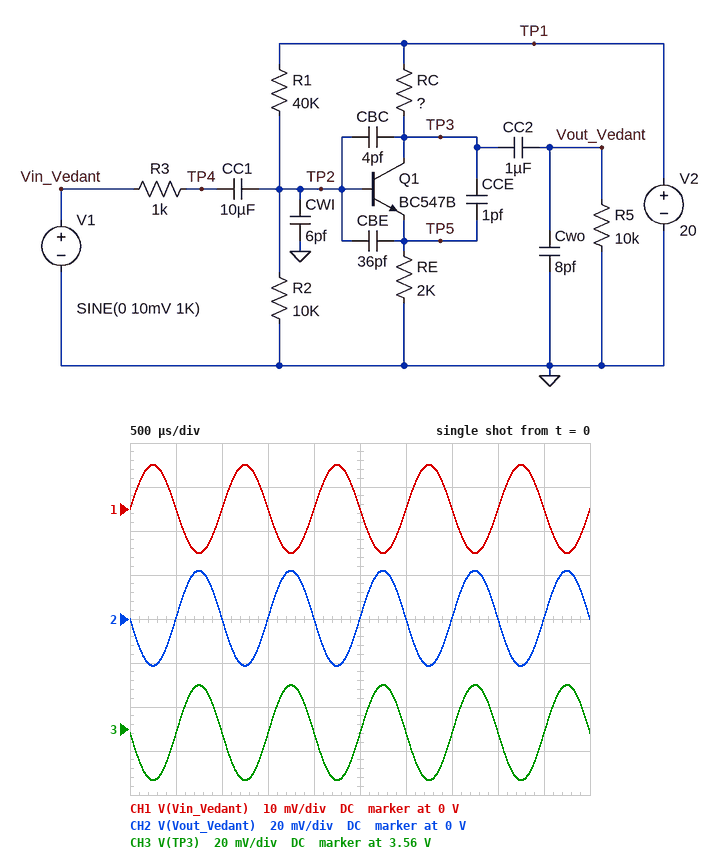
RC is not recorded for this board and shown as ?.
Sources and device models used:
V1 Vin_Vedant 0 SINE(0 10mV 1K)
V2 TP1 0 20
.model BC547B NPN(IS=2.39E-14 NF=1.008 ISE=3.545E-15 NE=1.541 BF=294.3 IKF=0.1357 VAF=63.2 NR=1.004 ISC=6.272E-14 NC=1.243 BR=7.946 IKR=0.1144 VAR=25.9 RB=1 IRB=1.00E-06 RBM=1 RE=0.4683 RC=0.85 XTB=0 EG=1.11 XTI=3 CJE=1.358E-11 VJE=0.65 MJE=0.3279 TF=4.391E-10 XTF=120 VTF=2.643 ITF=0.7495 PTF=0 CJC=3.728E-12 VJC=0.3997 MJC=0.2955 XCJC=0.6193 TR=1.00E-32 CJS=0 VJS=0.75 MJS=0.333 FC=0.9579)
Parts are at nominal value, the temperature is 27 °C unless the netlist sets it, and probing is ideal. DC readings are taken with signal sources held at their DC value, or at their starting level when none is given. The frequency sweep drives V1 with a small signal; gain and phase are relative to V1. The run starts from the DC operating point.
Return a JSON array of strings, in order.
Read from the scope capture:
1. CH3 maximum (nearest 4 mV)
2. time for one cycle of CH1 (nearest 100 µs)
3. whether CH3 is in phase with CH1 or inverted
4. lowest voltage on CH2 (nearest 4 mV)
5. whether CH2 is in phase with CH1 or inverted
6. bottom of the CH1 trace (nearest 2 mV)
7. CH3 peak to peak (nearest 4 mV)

["3.580 V", "1.0 ms", "inverted", "-20 mV", "inverted", "-10 mV", "44 mV"]
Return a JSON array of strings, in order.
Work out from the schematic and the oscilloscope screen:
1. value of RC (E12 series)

["10 kΩ"]
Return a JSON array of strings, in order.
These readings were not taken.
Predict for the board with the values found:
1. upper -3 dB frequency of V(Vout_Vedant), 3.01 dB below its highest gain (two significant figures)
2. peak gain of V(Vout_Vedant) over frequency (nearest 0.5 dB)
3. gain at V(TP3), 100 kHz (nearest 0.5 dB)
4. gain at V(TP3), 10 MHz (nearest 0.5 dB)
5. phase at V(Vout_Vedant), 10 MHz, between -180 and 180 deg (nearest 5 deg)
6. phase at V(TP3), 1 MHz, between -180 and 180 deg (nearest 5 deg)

["1.0 MHz", "6.5 dB", "6.5 dB", "-7.0 dB", "5 deg", "120 deg"]
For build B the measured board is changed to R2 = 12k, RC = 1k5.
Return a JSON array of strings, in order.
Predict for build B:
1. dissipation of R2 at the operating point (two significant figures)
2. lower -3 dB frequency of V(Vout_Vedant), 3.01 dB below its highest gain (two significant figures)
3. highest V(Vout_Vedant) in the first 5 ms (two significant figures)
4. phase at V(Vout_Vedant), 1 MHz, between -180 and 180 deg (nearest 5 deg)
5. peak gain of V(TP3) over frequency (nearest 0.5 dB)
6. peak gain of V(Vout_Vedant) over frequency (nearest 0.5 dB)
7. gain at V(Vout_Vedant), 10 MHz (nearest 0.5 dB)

["1.7 mW", "14 Hz", "5.9 mV", "165 deg", "-4.0 dB", "-4.5 dB", "-8.5 dB"]
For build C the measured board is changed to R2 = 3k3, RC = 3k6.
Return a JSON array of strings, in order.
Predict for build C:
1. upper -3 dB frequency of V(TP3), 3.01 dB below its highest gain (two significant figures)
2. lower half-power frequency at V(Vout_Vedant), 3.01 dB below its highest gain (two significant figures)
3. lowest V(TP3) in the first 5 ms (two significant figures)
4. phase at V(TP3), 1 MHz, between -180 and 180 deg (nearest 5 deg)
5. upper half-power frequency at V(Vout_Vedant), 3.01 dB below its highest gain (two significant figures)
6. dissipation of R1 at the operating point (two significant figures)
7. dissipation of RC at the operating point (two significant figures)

["2.9 MHz", "13 Hz", "18 V", "155 deg", "4.0 MHz", "8.5 mW", "740 µW"]
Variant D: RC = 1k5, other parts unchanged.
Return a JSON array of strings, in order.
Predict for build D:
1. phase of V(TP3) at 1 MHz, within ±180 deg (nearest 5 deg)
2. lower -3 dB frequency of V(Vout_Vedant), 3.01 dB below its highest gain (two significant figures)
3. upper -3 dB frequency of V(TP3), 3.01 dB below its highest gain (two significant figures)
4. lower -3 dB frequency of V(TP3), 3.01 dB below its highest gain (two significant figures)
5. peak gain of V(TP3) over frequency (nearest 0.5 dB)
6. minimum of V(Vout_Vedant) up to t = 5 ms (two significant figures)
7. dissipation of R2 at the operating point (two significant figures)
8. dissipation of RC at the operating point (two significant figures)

["165 deg", "14 Hz", "6.3 MHz", "1.6 Hz", "-4.0 dB", "-5.7 mV", "1.6 mW", "4.1 mW"]
